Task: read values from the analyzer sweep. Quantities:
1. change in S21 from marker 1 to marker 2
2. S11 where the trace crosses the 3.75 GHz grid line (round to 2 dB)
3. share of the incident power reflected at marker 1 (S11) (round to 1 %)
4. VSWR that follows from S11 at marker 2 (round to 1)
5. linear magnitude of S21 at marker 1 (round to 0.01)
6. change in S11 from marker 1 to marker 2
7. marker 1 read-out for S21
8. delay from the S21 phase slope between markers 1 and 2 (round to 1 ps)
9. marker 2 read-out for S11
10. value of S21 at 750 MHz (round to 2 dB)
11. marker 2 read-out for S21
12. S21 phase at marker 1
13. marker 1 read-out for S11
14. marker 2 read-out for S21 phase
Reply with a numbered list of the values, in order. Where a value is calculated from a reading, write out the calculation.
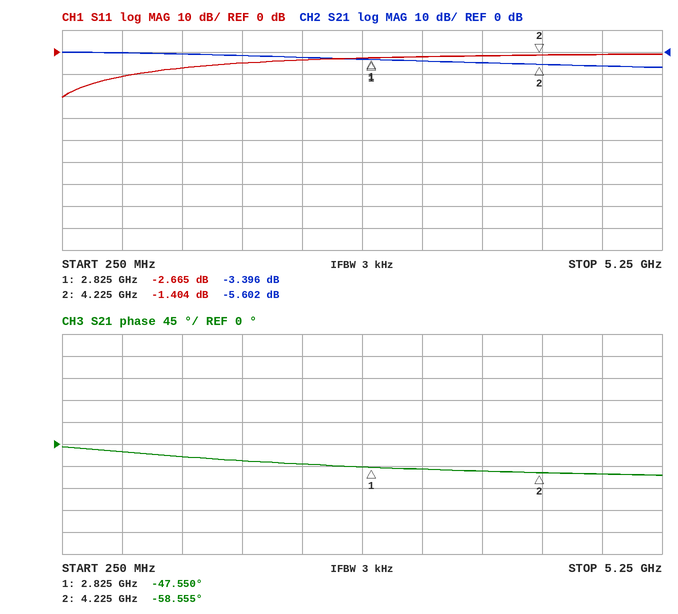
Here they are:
1. -5.602 − (-3.396) = -2.206 dB
2. -2 dB
3. 10^(-2.665/10) ≈ 54 %
4. (1 + 0.8507)/(1 − 0.8507) ≈ 12
5. 10^(-3.396/20) ≈ 0.68
6. -1.404 − (-2.665) = 1.261 dB
7. -3.396 dB
8. −(-58.555° − (-47.55°))/(360° × 1.4 GHz) ≈ 22 ps
9. -1.404 dB
10. 0 dB
11. -5.602 dB
12. -47.550°
13. -2.665 dB
14. -58.555°
